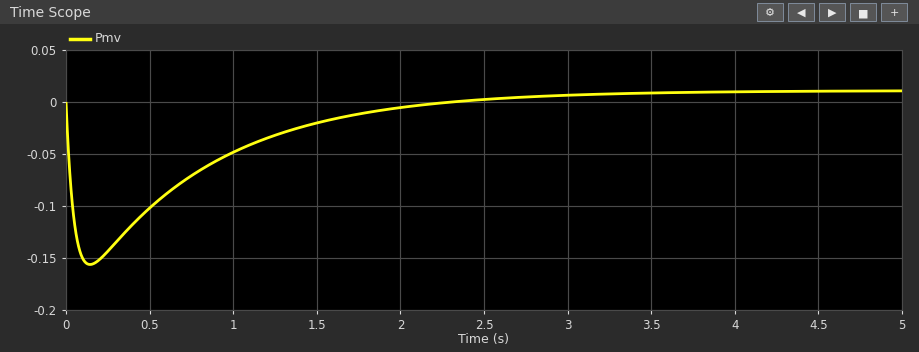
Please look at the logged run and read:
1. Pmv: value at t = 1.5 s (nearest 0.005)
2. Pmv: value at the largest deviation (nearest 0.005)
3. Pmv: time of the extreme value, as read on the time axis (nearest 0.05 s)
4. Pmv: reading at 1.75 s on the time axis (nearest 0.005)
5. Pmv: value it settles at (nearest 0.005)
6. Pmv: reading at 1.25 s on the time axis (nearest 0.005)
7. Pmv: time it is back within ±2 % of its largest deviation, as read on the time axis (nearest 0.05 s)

-0.020
-0.155
0.15 s
-0.010
0.010
-0.030
3.30 s
